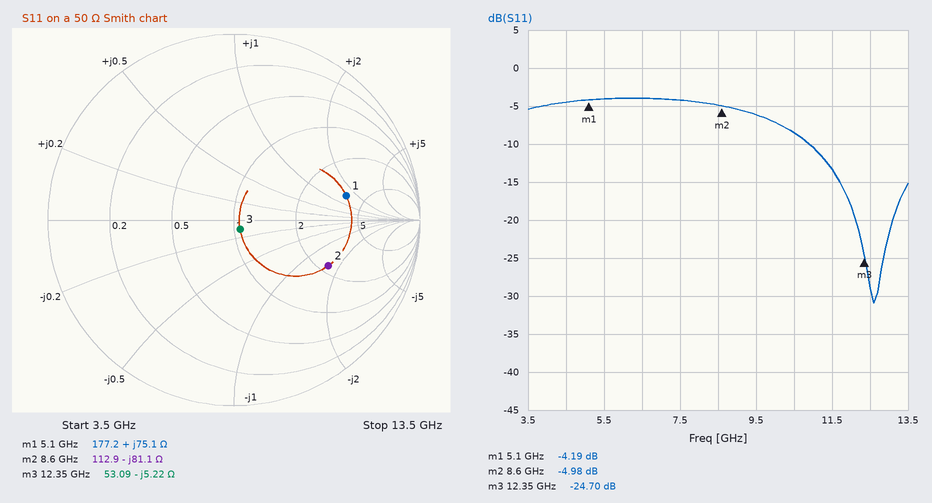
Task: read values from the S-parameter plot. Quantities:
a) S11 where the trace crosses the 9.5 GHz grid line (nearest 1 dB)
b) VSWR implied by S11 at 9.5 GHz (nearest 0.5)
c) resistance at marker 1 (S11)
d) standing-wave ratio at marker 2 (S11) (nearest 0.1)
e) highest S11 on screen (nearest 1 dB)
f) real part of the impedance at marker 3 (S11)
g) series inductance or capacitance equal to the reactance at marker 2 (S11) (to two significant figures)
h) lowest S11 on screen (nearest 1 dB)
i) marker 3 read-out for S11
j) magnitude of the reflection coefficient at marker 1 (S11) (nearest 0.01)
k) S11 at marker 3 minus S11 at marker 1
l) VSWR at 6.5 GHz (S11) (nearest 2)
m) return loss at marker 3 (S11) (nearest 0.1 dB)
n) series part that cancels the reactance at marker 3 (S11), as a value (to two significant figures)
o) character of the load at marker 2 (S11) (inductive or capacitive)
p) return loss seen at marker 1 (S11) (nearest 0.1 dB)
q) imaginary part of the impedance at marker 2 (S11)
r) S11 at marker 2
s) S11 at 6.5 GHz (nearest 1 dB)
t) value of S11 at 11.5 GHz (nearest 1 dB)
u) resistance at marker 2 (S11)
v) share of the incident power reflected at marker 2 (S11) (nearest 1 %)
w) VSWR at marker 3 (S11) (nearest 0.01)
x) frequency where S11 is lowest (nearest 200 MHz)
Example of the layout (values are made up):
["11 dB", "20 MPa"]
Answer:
["-6 dB", "3.0", "177.2 Ω", "3.6", "-4 dB", "53.09 Ω", "230 fF", "-31 dB", "-24.70 dB", "0.62", "-20.51 dB", "4", "24.6 dB", "67 pH", "capacitive", "4.2 dB", "-81.1 Ω", "-4.98 dB", "-4 dB", "-13 dB", "112.9 Ω", "32 %", "1.12", "12.6 GHz"]
